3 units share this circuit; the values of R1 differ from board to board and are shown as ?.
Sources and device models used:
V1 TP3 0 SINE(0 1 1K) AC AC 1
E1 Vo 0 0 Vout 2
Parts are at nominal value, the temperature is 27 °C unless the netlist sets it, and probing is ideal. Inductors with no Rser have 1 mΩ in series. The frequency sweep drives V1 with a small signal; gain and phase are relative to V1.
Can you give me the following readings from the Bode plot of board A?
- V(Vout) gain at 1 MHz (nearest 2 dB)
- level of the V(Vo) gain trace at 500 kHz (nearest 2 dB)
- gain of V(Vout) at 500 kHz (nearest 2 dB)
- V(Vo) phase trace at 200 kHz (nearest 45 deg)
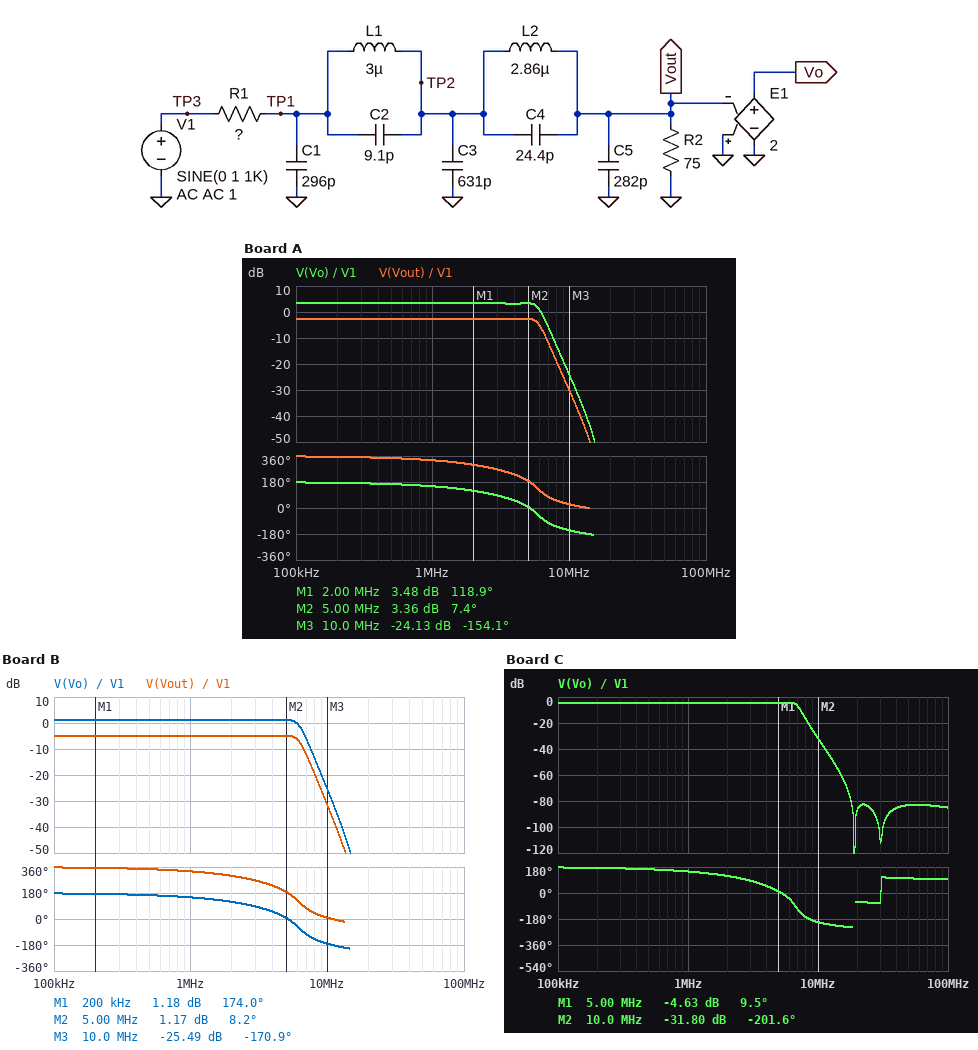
-2 dB
4 dB
-2 dB
180 deg
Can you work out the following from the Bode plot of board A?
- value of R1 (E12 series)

27 Ω
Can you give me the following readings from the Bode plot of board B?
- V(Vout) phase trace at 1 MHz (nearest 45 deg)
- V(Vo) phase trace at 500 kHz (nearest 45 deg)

315 deg
180 deg
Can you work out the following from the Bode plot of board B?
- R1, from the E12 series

56 Ω
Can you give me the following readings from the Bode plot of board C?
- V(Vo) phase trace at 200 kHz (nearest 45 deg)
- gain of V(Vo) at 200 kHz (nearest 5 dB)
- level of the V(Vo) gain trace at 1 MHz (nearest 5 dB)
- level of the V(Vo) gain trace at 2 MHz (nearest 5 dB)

180 deg
-5 dB
-5 dB
-5 dB
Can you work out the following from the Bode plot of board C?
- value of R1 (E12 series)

180 Ω
